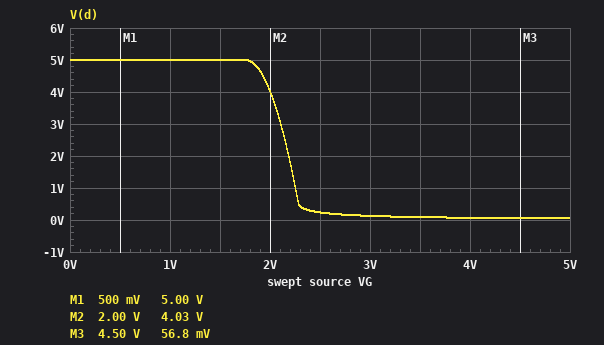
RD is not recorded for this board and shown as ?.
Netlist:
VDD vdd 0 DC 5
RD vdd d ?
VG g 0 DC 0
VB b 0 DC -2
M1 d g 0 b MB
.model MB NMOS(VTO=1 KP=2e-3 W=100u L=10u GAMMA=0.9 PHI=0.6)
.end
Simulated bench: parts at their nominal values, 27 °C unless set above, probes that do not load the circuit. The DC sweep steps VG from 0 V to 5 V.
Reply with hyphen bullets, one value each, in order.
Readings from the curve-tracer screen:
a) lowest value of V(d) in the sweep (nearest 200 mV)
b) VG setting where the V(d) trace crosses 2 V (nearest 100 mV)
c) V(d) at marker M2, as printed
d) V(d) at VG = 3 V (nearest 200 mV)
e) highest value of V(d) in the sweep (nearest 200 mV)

- 0 V
- 2.2 V
- 4.03 V
- 200 mV
- 5.0 V
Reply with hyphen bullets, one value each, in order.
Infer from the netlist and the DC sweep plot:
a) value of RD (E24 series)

- 1.6 kΩ
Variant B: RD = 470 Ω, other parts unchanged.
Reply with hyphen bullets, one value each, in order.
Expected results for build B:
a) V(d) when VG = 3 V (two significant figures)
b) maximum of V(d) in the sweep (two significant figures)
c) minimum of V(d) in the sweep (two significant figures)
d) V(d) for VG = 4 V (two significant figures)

- 480 mV
- 5.0 V
- 160 mV
- 240 mV
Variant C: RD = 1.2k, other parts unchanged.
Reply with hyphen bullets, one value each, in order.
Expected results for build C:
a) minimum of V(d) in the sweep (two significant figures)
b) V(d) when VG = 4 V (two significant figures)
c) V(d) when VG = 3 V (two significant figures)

- 64 mV
- 93 mV
- 170 mV
